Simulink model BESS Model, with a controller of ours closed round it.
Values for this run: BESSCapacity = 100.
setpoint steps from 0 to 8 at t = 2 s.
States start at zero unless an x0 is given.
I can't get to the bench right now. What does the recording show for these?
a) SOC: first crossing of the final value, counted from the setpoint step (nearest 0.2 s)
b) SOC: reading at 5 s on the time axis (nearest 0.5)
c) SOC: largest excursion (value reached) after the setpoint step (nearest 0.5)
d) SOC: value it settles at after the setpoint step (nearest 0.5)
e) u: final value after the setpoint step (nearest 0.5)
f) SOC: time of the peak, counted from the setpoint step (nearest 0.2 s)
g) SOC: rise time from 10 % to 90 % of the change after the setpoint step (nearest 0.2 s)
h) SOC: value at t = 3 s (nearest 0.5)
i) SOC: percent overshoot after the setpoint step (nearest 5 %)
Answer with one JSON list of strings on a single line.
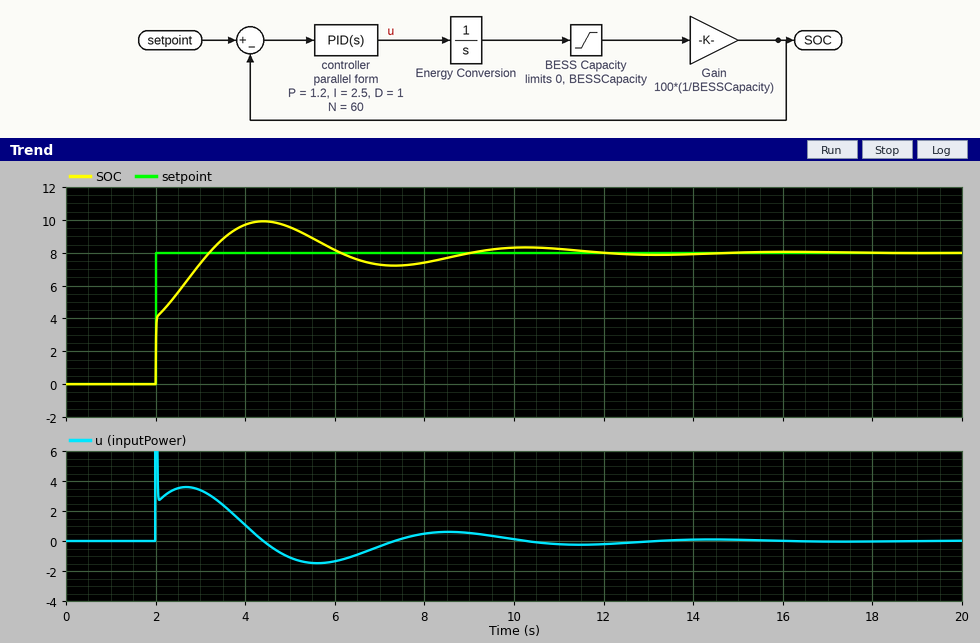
["1.2 s", "9.5", "10.0", "8.0", "0.0", "2.4 s", "1.0 s", "7.5", "25 %"]
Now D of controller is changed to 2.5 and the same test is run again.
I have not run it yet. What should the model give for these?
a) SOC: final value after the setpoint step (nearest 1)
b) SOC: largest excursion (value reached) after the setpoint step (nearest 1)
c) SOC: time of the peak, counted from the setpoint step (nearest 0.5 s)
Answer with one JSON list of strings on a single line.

["8", "9", "3.5 s"]
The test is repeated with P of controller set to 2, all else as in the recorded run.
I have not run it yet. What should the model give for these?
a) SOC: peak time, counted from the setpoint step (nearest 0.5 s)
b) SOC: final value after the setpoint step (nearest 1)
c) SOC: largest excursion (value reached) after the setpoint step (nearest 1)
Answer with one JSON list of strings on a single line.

["2.0 s", "8", "9"]
